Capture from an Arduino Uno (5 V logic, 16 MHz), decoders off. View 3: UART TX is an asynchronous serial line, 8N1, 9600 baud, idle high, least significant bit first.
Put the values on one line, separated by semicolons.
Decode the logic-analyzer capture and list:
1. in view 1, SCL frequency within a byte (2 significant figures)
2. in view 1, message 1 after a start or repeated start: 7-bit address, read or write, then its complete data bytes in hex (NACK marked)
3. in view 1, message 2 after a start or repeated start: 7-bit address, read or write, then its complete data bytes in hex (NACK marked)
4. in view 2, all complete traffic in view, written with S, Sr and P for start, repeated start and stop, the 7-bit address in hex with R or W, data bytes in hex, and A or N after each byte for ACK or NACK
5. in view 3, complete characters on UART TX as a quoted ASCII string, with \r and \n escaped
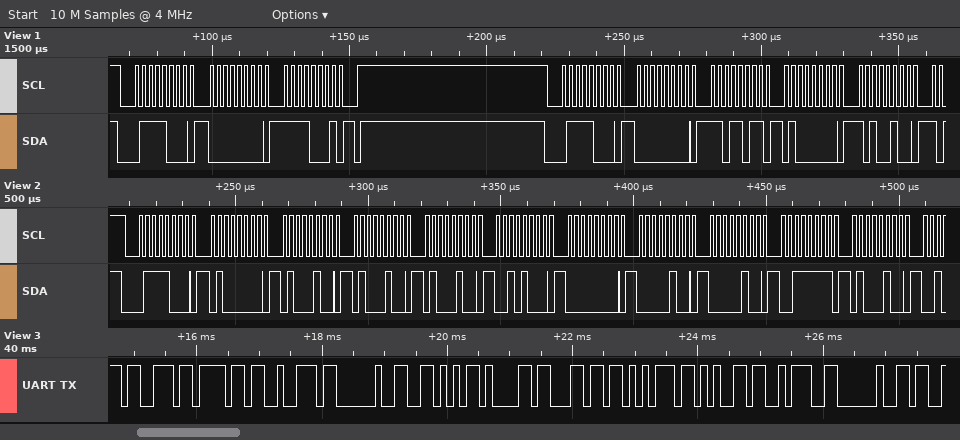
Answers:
400 kHz; 0x3C write: 00 F1; 0x3C write: 00 DB 40 A4; S 3CW A 40 A 44 A 44 A 44 A 28 A 00 A 04 A 04 A 3F A 44 A; "sor Value: "
